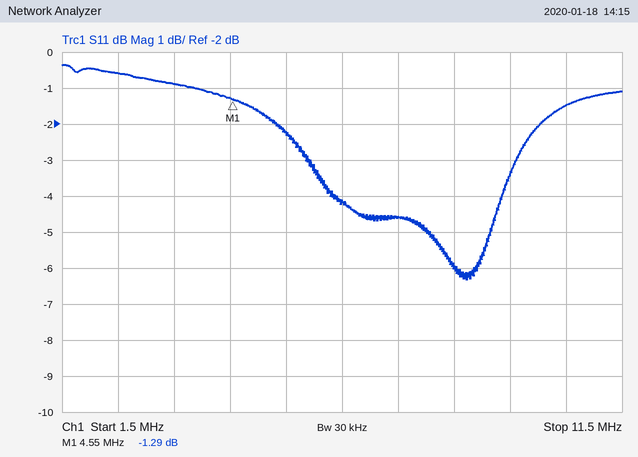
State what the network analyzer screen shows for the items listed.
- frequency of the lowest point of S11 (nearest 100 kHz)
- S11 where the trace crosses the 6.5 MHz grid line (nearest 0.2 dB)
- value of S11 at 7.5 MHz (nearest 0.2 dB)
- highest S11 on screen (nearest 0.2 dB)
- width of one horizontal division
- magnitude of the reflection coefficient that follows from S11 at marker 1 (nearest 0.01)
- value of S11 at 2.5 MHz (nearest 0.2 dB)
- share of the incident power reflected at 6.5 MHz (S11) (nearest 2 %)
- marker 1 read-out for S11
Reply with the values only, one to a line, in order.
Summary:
8.7 MHz
-4.2 dB
-4.6 dB
-0.4 dB
1 MHz
0.86
-0.6 dB
38 %
-1.29 dB
